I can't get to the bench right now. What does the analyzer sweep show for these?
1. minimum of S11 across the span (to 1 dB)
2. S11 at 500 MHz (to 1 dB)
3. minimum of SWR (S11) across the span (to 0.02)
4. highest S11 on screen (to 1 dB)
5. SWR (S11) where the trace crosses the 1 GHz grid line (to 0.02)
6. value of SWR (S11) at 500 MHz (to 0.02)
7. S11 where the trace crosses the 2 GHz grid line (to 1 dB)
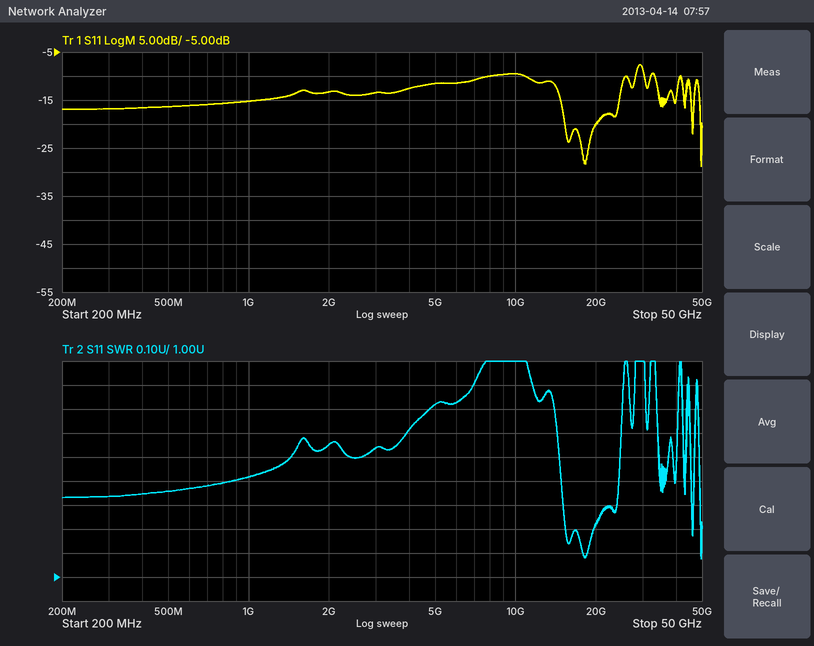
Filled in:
-29 dB
-16 dB
1.08
-8 dB
1.42
1.36
-13 dB
